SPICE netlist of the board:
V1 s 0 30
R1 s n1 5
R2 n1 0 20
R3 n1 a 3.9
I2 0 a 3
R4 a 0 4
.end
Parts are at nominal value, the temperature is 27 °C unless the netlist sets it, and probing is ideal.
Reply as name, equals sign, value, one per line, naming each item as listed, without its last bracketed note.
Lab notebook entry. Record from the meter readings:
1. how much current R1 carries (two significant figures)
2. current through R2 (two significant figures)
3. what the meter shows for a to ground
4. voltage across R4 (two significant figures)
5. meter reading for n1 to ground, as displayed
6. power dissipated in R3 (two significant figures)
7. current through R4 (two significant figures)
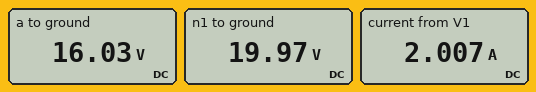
how much current R1 carries = 2.0 A
current through R2 = 1.0 A
what the meter shows for a to ground = 16.03 V
voltage across R4 = 16 V
meter reading for n1 to ground, as displayed = 19.97 V
power dissipated in R3 = 4.0 W
current through R4 = 4.0 A
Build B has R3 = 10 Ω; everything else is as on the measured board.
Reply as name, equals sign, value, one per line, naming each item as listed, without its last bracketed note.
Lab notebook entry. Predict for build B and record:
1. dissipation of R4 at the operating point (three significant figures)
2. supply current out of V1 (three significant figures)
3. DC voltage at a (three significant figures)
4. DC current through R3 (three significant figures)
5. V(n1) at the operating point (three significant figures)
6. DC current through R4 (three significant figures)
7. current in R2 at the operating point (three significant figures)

dissipation of R4 at the operating point = 53.8 W
supply current out of V1 = 1.73 A
DC voltage at a = 14.7 V
DC current through R3 = 667 mA
V(n1) at the operating point = 21.3 V
DC current through R4 = 3.67 A
current in R2 at the operating point = 1.07 A
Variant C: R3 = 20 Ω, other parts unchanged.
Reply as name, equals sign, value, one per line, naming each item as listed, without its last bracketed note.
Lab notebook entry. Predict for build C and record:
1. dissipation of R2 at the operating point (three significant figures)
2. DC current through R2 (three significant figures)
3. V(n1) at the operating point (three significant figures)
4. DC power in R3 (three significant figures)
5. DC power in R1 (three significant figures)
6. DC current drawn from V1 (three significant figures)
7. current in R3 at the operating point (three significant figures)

dissipation of R2 at the operating point = 24.8 W
DC current through R2 = 1.11 A
V(n1) at the operating point = 22.3 V
DC power in R3 = 3.67 W
DC power in R1 = 11.9 W
DC current drawn from V1 = 1.54 A
current in R3 at the operating point = 429 mA
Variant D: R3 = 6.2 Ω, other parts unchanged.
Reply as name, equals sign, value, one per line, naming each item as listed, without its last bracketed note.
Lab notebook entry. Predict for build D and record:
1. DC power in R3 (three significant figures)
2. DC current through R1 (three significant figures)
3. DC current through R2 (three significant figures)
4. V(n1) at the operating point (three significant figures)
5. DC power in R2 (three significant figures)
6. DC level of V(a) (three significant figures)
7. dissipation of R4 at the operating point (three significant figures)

DC power in R3 = 4.43 W
DC current through R1 = 1.88 A
DC current through R2 = 1.03 A
V(n1) at the operating point = 20.6 V
DC power in R2 = 21.3 W
DC level of V(a) = 15.4 V
dissipation of R4 at the operating point = 59.1 W
